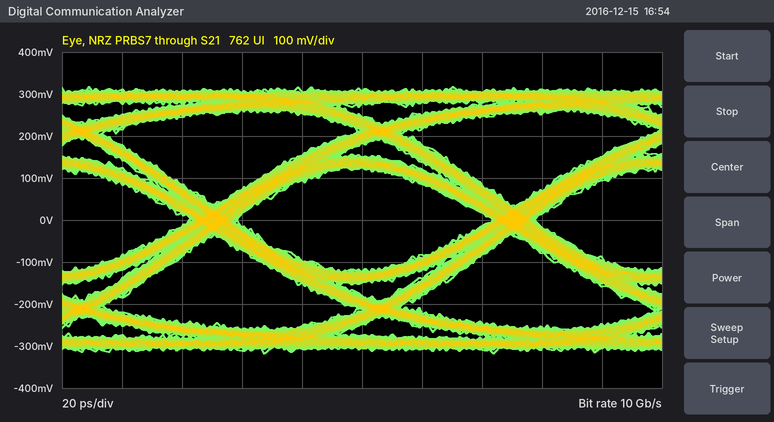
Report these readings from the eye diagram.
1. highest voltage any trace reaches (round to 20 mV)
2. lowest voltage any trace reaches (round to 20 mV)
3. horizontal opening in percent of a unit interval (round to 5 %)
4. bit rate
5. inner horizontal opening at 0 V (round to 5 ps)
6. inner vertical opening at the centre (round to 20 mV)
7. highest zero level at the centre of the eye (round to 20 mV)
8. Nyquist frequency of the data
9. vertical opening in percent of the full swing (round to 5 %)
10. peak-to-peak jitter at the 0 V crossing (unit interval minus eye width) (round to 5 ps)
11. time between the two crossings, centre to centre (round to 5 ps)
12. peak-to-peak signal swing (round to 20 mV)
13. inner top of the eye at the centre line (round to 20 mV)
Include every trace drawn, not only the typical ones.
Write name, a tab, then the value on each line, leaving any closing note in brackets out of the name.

highest voltage any trace reaches	320 mV
lowest voltage any trace reaches	-320 mV
horizontal opening in percent of a unit interval	85 %
bit rate	10 Gb/s
inner horizontal opening at 0 V	85 ps
inner vertical opening at the centre	240 mV
highest zero level at the centre of the eye	-120 mV
Nyquist frequency of the data	5 GHz
vertical opening in percent of the full swing	40 %
peak-to-peak jitter at the 0 V crossing (unit interval minus eye width)	15 ps
time between the two crossings, centre to centre	100 ps
peak-to-peak signal swing	640 mV
inner top of the eye at the centre line	120 mV
